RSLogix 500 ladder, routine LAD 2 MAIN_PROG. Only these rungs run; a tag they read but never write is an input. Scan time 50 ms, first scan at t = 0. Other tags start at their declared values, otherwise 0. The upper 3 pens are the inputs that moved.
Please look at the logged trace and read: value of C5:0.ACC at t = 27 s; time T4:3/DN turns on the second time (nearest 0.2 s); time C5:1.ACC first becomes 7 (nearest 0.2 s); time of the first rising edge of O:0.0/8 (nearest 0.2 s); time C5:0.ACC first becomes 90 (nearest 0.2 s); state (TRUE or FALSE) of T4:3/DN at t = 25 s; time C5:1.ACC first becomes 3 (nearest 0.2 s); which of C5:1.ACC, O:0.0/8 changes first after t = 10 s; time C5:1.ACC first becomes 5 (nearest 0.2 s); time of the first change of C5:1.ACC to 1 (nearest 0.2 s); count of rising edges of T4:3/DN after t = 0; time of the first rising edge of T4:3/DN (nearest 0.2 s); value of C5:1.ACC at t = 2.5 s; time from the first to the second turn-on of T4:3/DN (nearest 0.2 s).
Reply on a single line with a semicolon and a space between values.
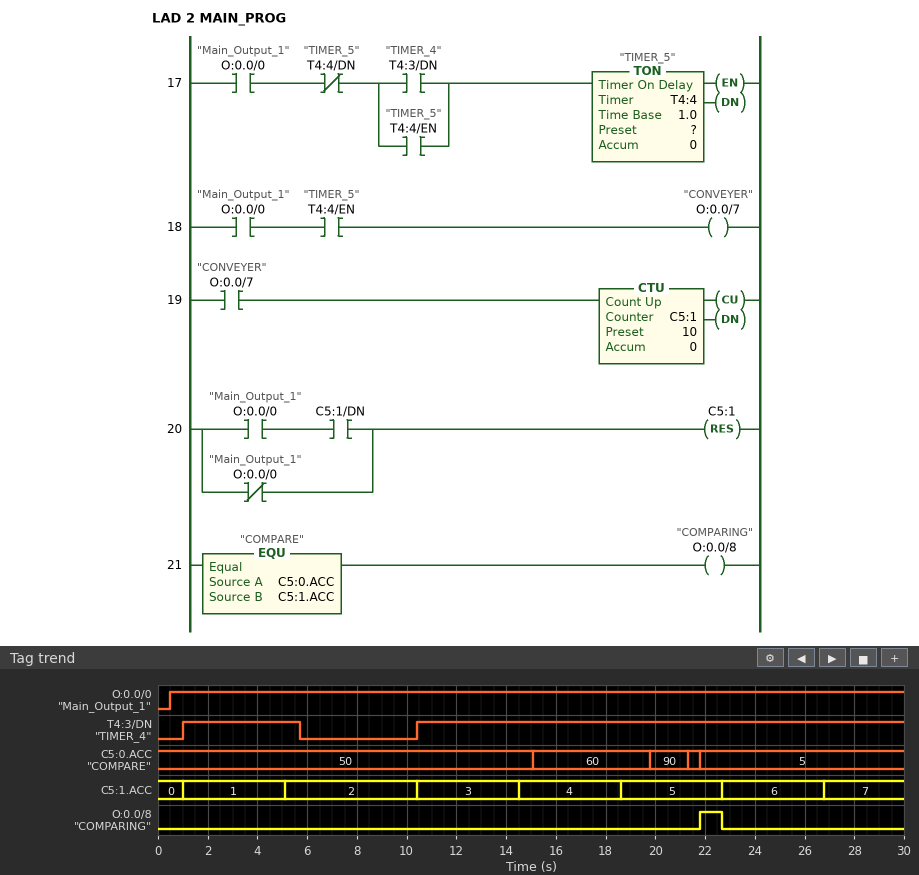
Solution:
5; 10.4 s; 26.8 s; 21.8 s; 19.8 s; TRUE; 10.4 s; C5:1.ACC; 18.6 s; 1.0 s; 2; 1.0 s; 1; 9.4 s
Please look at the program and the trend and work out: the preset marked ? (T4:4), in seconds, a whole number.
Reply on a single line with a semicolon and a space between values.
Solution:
4 s
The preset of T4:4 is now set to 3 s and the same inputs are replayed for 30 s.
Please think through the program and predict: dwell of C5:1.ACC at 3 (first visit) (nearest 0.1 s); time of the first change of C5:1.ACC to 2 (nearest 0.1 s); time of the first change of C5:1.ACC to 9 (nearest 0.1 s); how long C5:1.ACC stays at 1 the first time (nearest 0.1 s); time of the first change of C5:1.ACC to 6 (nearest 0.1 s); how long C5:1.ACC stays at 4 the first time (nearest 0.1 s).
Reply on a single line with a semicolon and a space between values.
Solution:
3.1 s; 4.1 s; 29.0 s; 3.1 s; 19.7 s; 3.1 s
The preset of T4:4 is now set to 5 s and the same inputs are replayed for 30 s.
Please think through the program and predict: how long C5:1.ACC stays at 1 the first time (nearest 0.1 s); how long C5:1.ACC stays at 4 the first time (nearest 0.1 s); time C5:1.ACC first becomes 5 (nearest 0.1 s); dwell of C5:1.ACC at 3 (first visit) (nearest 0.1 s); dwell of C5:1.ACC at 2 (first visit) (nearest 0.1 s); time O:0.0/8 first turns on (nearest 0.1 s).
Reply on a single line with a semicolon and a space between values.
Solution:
9.4 s; 5.1 s; 25.7 s; 5.1 s; 5.1 s; 25.7 s
